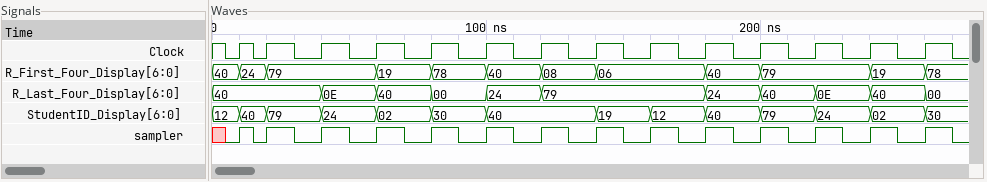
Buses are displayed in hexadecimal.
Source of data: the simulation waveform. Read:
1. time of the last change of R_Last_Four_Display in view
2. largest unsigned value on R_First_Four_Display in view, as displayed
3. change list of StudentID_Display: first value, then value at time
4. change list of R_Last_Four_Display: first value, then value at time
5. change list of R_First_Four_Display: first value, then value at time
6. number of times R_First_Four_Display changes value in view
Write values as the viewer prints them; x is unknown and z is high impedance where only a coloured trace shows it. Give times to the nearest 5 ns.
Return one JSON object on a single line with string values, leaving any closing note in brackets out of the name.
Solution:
{"time of the last change of R_Last_Four_Display in view": "260 ns", "largest unsigned value on R_First_Four_Display in view, as displayed": "79", "change list of StudentID_Display: first value, then value at time": "12, 40 at 10 ns, 79 at 20 ns, 24 at 40 ns, 02 at 60 ns, 30 at 80 ns, 40 at 100 ns, 19 at 140 ns, 12 at 160 ns, 40 at 180 ns, 79 at 200 ns, 24 at 220 ns, 02 at 240 ns, 30 at 260 ns", "change list of R_Last_Four_Display: first value, then value at time": "40, 0E at 40 ns, 40 at 60 ns, 00 at 80 ns, 24 at 100 ns, 79 at 120 ns, 24 at 180 ns, 40 at 200 ns, 0E at 220 ns, 40 at 240 ns, 00 at 260 ns", "change list of R_First_Four_Display: first value, then value at time": "40, 24 at 10 ns, 79 at 20 ns, 19 at 60 ns, 78 at 80 ns, 40 at 100 ns, 08 at 120 ns, 06 at 140 ns, 40 at 180 ns, 79 at 200 ns, 19 at 240 ns, 78 at 260 ns", "number of times R_First_Four_Display changes value in view": "11"}
